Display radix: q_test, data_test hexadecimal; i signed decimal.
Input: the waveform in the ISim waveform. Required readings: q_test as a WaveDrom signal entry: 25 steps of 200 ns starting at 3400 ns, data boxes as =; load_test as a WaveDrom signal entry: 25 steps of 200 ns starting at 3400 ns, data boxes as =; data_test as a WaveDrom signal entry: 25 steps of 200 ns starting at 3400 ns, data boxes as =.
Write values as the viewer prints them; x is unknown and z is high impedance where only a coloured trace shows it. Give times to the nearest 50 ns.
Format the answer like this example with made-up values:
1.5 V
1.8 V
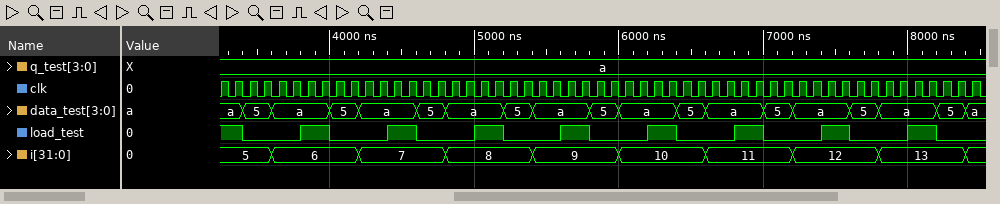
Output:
{name: 'q_test', wave: '=........................', data: 'a'}
{name: 'load_test', wave: '0.10.10.10.10.10.10.10.10'}
{name: 'data_test', wave: '==.==.==.==.==.==.==.==.=', data: '5 a 5 a 5 a 5 a 5 a 5 a 5 a 5 a 5'}
